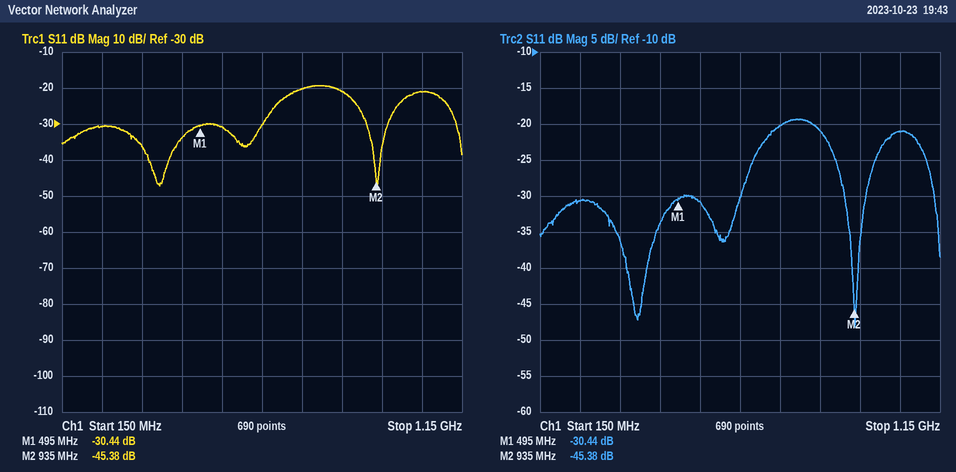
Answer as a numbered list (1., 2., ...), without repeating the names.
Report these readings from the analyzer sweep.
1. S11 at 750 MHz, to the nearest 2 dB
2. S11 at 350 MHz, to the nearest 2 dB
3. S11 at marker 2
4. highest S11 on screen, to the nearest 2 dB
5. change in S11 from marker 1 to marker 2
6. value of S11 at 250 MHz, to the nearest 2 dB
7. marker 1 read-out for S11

1. -20 dB
2. -36 dB
3. -45.38 dB
4. -20 dB
5. -14.94 dB
6. -30 dB
7. -30.44 dB
